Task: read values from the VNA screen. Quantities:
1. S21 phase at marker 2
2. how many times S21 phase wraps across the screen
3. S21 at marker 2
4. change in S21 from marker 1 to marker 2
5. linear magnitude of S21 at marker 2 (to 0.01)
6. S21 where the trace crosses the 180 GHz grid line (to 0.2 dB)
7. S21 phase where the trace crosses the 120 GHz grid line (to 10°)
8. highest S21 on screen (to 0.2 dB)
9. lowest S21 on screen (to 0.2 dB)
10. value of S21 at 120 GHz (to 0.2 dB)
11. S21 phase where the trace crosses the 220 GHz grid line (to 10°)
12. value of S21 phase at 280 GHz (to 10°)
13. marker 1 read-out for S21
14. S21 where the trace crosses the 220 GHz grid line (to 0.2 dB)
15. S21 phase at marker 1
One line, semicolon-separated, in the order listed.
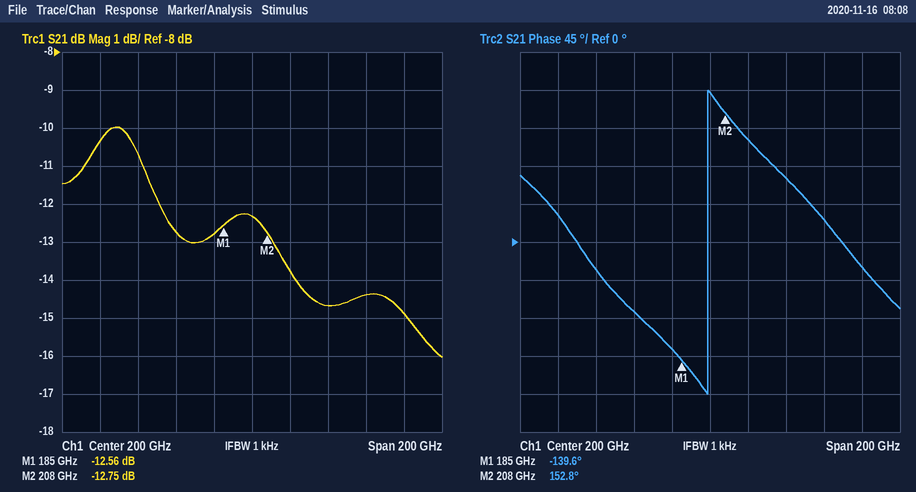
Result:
152.8°; 1; -12.75 dB; -0.19 dB; 0.23; -12.8 dB; 30°; -10.0 dB; -16.0 dB; -10.4 dB; 120°; -30°; -12.56 dB; -13.8 dB; -139.6°
